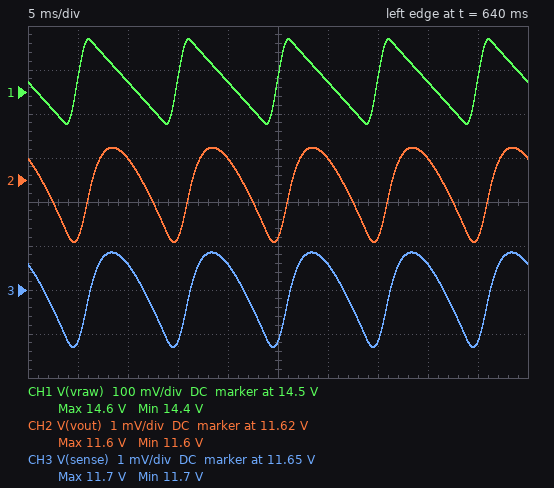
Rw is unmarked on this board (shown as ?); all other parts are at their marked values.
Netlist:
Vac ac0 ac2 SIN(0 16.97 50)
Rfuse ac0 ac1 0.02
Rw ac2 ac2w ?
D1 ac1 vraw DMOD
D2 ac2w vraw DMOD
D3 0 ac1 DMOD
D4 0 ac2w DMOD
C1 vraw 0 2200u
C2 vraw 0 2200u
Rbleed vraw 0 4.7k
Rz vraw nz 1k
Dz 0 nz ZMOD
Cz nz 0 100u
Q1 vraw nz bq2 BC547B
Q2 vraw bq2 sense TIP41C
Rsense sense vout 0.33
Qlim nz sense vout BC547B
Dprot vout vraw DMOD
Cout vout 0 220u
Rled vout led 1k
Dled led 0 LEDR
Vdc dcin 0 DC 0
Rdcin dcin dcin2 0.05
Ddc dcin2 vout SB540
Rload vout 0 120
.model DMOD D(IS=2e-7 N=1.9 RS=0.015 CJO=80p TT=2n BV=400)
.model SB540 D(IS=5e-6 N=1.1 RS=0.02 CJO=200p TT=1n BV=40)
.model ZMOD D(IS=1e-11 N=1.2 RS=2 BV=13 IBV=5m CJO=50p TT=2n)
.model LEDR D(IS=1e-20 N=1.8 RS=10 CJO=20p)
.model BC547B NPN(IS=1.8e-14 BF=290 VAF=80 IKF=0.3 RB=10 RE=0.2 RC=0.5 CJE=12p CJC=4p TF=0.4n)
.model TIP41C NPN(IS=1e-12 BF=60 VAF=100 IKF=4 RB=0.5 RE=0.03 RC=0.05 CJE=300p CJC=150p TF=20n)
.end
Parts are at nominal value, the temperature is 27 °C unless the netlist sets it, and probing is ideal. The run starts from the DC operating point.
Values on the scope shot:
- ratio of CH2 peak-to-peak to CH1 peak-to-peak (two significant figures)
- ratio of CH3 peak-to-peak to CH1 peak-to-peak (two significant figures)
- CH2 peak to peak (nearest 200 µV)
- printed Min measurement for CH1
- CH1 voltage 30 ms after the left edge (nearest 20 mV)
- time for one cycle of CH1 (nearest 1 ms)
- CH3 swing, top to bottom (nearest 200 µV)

0.011
0.011
2.2 mV
14.4 V
14.52 V
10 ms
2.2 mV
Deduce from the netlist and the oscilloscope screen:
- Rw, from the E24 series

1.3 Ω
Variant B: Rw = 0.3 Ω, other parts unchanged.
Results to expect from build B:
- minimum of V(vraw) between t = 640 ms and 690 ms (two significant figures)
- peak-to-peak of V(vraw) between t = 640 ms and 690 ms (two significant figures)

15 V
210 mV
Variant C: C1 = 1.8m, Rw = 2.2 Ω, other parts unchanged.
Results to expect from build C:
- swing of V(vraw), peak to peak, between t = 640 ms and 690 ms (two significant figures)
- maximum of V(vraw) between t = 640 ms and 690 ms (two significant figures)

200 mV
14 V
